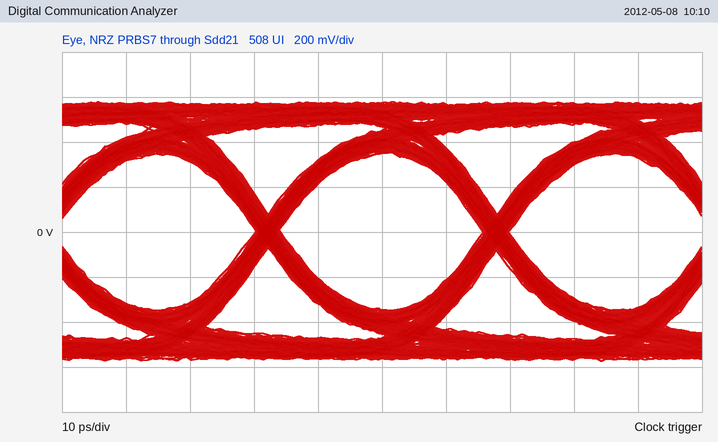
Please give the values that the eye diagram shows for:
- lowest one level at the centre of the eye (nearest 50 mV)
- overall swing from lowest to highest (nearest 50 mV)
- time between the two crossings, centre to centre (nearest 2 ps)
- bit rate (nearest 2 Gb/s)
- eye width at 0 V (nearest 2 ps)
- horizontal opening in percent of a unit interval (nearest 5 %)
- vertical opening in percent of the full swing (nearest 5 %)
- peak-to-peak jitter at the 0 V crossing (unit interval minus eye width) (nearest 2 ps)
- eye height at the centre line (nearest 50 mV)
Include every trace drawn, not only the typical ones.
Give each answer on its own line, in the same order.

350 mV
1.15 V
36 ps
28 Gb/s
32 ps
90 %
60 %
4 ps
700 mV
